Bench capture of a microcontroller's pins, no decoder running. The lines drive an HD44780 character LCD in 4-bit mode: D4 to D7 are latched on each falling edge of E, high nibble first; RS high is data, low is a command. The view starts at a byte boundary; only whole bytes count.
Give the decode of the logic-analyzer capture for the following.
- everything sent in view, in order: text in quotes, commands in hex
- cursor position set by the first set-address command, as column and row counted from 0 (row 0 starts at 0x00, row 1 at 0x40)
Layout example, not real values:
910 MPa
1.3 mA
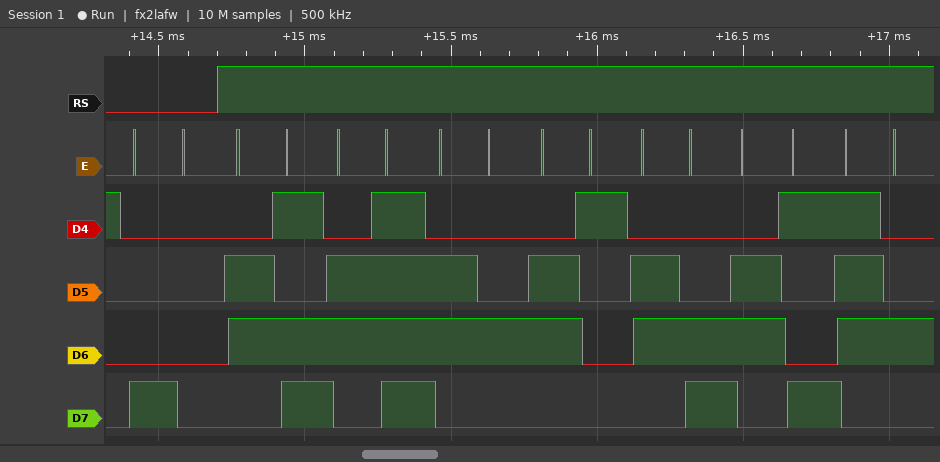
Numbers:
0x80 "modalit"
column 0, row 0
